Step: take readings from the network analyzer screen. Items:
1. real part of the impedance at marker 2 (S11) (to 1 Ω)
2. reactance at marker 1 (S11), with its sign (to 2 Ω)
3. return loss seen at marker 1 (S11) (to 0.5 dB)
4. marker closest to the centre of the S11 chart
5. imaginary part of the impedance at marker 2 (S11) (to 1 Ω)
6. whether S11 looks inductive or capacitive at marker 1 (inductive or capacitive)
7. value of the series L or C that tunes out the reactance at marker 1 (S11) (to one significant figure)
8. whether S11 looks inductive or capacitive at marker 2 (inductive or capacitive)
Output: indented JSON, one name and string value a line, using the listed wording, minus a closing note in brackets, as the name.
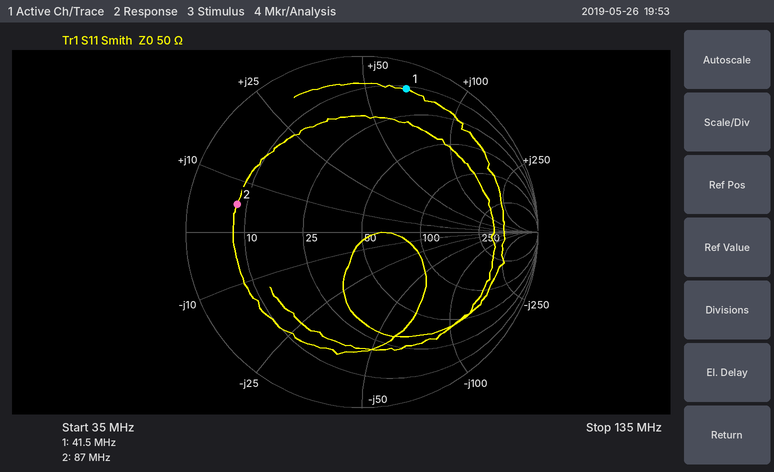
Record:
{
  "real part of the impedance at marker 2 (S11)": "8 Ω",
  "reactance at marker 1 (S11), with its sign": "+66 Ω",
  "return loss seen at marker 1 (S11)": "1.5 dB",
  "marker closest to the centre of the S11 chart": "marker 2",
  "imaginary part of the impedance at marker 2 (S11)": "+5 Ω",
  "whether S11 looks inductive or capacitive at marker 1": "inductive",
  "value of the series L or C that tunes out the reactance at marker 1 (S11)": "60 pF",
  "whether S11 looks inductive or capacitive at marker 2": "inductive"
}
